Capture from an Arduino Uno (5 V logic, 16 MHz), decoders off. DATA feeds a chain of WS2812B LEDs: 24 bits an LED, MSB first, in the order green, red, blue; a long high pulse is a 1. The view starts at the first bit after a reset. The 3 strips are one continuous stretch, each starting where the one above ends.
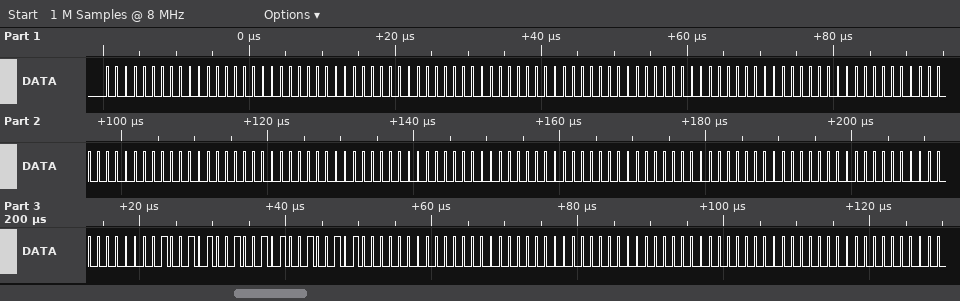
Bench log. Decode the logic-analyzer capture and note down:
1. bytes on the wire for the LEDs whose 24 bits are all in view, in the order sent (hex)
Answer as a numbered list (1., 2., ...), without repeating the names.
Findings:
1. 00 00 00 00 00 00 00 00 00 00 00 00 00 00 00 00 00 00 00 00 00 00 00 00 25 25 25 00 00 00 00 00 00
